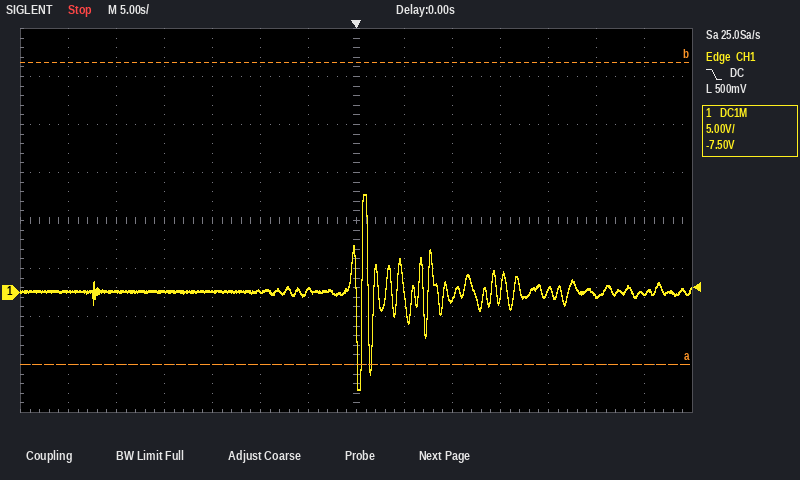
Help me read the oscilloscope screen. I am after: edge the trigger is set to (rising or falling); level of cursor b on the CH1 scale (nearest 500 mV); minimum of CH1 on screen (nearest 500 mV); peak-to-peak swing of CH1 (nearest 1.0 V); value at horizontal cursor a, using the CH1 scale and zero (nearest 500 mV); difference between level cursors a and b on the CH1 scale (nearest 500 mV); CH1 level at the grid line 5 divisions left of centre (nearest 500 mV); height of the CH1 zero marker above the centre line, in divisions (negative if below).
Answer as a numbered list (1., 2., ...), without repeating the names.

1. falling
2. 24.0 V
3. -10.0 V
4. 20.0 V
5. -7.5 V
6. 31.5 V
7. 0.0 V
8. -1.5 div
